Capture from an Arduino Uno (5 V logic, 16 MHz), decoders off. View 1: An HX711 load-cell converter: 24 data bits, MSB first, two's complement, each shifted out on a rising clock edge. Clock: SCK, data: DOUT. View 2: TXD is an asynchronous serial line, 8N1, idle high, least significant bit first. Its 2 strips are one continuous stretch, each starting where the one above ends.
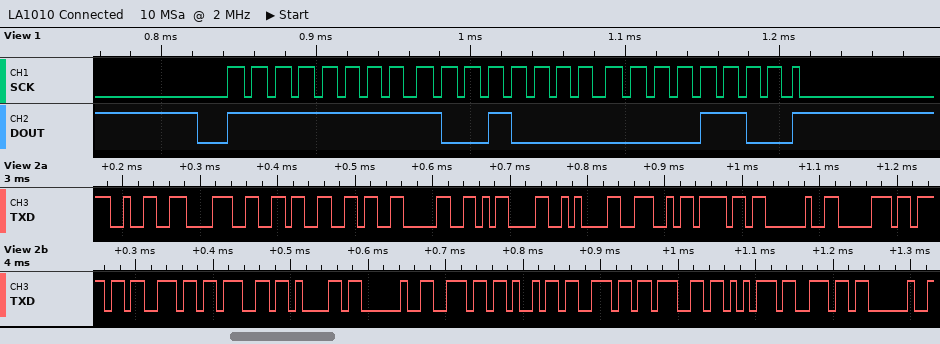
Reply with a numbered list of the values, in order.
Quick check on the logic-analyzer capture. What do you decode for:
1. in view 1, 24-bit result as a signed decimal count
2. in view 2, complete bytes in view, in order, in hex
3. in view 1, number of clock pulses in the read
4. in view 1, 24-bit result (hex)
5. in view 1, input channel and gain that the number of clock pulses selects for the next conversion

1. -28660
2. 0x32 0x38 0x36 0x36 0x30 0x0D 0x0A 0x4E 0x6F 0x20 0x70 0x6F 0x6E 0x67 0x61 0x20 0x6E 0x69 0x6E 0x67 0x75 0x6E 0x20
3. 25
4. 0xFF900C
5. channel A, gain 128
